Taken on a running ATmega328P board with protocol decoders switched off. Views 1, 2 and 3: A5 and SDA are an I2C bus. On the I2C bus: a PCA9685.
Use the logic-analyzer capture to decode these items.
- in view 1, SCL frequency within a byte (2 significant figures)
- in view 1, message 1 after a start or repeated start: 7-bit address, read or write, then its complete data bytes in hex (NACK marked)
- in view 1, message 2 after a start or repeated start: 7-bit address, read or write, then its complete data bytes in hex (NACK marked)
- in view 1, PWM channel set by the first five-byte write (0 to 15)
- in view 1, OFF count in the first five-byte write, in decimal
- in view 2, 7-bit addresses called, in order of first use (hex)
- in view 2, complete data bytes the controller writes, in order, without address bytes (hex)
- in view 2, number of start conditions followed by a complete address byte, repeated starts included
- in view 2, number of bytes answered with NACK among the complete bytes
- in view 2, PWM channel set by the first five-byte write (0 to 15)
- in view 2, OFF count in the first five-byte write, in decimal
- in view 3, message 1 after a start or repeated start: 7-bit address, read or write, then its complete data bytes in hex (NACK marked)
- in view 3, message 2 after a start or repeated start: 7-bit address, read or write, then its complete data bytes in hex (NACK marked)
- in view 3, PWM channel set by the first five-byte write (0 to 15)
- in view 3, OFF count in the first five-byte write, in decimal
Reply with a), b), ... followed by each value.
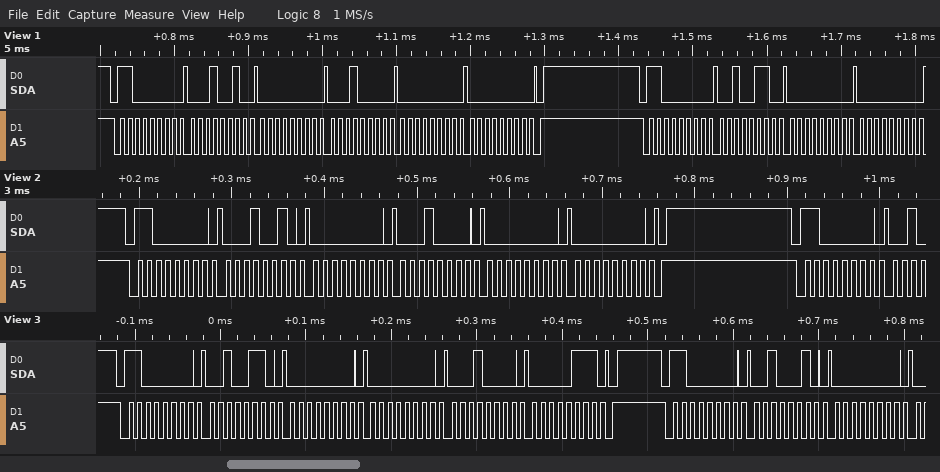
a) 100 kHz
b) 0x60 write: 12 00 10 00 00
c) 0x60 write: 26 00 00
d) 3
e) 0
f) 0x60
g) 12 00 10 00 00
h) 2
i) 0
j) 3
k) 0
l) 0x60 write: 26 00 00 10 07
m) 0x60 write: 22 00
n) 8
o) 1808
